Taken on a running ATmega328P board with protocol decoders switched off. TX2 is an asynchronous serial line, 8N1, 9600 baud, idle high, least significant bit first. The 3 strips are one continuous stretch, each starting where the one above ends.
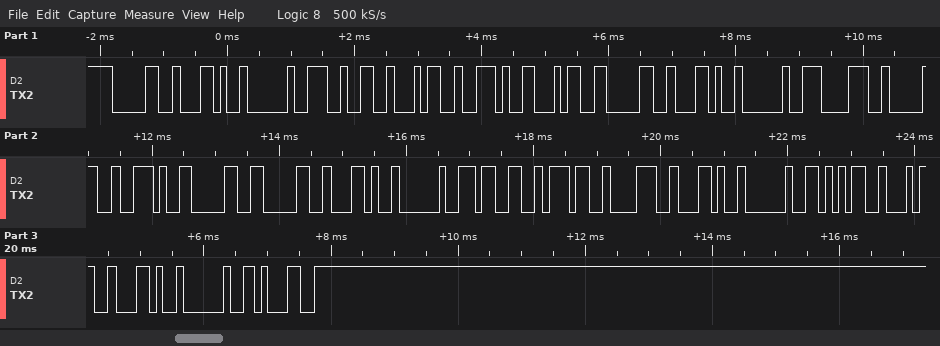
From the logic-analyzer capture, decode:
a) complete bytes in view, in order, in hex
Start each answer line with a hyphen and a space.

- 30 2C 20 32 34 2E 34 30 2C 20 38 30 2E 30 30 2C 20 33 37 38 2C 20 35 34 2C 20 31
